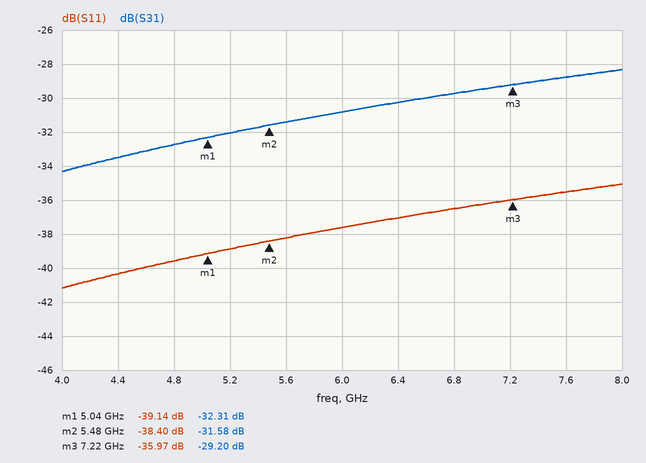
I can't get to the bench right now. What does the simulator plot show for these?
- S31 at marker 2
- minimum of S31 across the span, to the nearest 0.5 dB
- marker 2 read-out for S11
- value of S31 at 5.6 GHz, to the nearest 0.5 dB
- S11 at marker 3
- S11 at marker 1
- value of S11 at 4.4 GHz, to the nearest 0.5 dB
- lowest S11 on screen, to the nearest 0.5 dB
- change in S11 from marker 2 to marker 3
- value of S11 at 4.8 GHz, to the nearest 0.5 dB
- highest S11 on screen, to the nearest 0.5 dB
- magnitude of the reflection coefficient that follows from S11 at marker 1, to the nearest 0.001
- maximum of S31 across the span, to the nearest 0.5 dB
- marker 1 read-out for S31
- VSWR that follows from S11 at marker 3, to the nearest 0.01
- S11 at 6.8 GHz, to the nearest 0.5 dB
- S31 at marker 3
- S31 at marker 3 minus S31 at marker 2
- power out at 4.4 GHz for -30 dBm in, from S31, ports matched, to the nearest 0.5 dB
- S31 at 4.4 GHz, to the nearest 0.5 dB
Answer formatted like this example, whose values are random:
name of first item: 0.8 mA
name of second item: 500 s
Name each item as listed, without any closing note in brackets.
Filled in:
S31 at marker 2: -31.58 dB
minimum of S31 across the span, to the nearest 0.5 dB: -34.5 dB
marker 2 read-out for S11: -38.40 dB
value of S31 at 5.6 GHz, to the nearest 0.5 dB: -31.5 dB
S11 at marker 3: -35.97 dB
S11 at marker 1: -39.14 dB
value of S11 at 4.4 GHz, to the nearest 0.5 dB: -40.5 dB
lowest S11 on screen, to the nearest 0.5 dB: -41.0 dB
change in S11 from marker 2 to marker 3: 2.43 dB
value of S11 at 4.8 GHz, to the nearest 0.5 dB: -39.5 dB
highest S11 on screen, to the nearest 0.5 dB: -35.0 dB
magnitude of the reflection coefficient that follows from S11 at marker 1, to the nearest 0.001: 0.011
maximum of S31 across the span, to the nearest 0.5 dB: -28.5 dB
marker 1 read-out for S31: -32.31 dB
VSWR that follows from S11 at marker 3, to the nearest 0.01: 1.03
S11 at 6.8 GHz, to the nearest 0.5 dB: -36.5 dB
S31 at marker 3: -29.20 dB
S31 at marker 3 minus S31 at marker 2: 2.38 dB
power out at 4.4 GHz for -30 dBm in, from S31, ports matched, to the nearest 0.5 dB: -63.5 dBm
S31 at 4.4 GHz, to the nearest 0.5 dB: -33.5 dB
